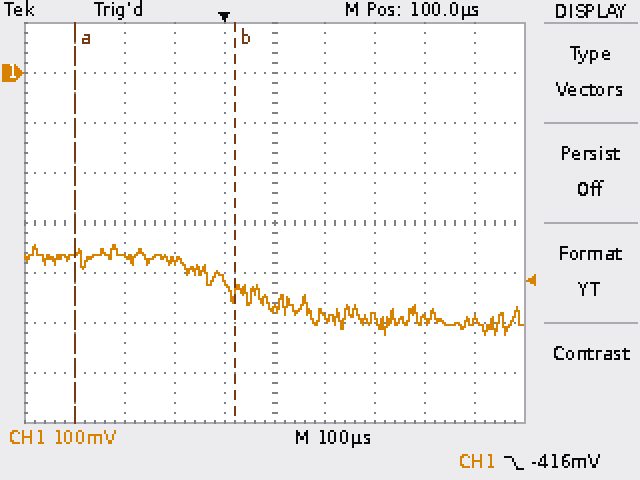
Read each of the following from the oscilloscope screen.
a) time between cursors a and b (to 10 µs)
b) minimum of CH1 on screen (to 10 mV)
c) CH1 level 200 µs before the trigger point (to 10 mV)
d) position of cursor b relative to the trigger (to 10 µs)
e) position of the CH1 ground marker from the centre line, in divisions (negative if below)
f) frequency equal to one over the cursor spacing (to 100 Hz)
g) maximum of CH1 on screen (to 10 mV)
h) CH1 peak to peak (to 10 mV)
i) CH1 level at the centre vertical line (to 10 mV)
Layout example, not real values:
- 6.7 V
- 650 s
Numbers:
- 320 µs
- -520 mV
- -370 mV
- +20 µs
- +3.0 div
- 3.1 kHz
- -340 mV
- 180 mV
- -470 mV
